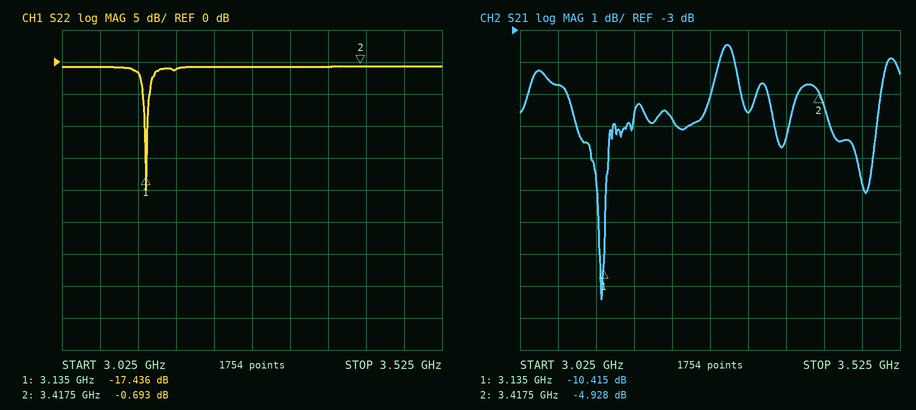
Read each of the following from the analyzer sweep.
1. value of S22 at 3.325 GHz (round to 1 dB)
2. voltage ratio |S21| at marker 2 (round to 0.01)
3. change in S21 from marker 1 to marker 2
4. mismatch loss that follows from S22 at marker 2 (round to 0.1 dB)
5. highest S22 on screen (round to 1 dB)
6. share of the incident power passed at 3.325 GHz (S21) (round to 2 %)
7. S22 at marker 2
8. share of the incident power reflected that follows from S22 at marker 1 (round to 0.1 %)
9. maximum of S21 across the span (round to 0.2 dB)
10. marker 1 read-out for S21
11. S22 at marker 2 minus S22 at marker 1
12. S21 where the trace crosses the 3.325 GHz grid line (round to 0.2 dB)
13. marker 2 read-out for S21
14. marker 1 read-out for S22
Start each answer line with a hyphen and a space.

- -1 dB
- 0.57
- 5.487 dB
- 8.3 dB
- -1 dB
- 28 %
- -0.693 dB
- 1.8 %
- -3.4 dB
- -10.415 dB
- 16.743 dB
- -5.6 dB
- -4.928 dB
- -17.436 dB
